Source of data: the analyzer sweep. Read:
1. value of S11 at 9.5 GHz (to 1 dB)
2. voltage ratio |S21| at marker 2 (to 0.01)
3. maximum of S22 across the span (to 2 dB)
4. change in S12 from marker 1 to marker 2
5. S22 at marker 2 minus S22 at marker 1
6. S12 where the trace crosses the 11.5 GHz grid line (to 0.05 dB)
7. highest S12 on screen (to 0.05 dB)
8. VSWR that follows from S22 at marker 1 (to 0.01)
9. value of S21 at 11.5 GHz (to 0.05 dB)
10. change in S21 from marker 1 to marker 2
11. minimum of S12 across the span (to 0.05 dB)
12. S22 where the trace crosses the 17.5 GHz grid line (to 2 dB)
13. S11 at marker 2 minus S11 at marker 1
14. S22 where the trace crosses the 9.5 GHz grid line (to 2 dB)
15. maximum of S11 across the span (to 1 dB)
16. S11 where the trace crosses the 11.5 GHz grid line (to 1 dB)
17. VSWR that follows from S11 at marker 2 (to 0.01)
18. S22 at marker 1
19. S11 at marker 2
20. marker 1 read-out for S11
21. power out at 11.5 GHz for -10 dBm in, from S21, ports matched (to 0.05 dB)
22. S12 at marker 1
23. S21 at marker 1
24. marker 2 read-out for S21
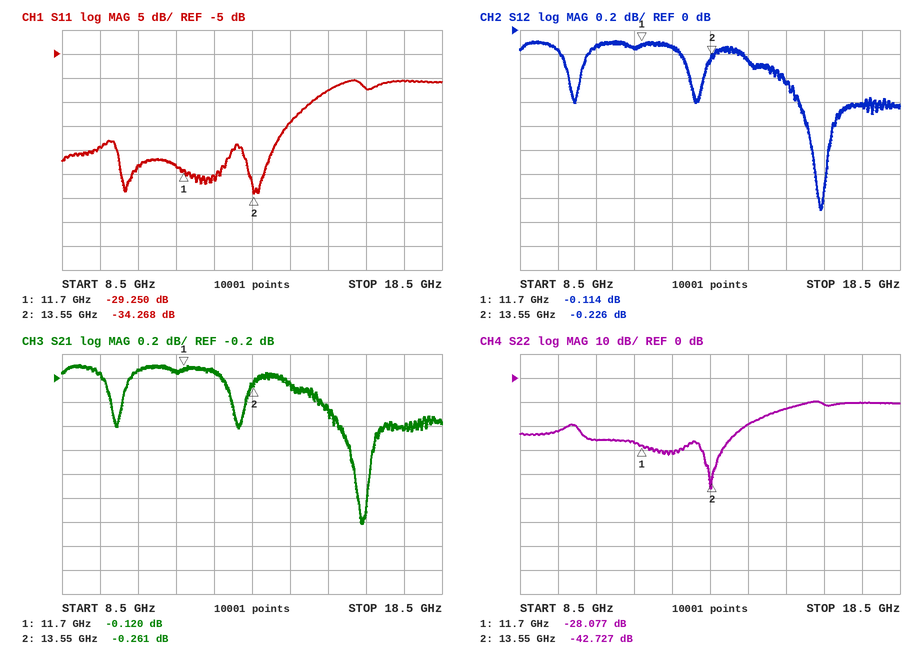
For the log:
-24 dB
0.97
-10 dB
-0.112 dB
-14.650 dB
-0.15 dB
-0.10 dB
1.08
-0.15 dB
-0.141 dB
-1.50 dB
-10 dB
-5.018 dB
-22 dB
-10 dB
-28 dB
1.04
-28.077 dB
-34.268 dB
-29.250 dB
-10.15 dBm
-0.114 dB
-0.120 dB
-0.261 dB
